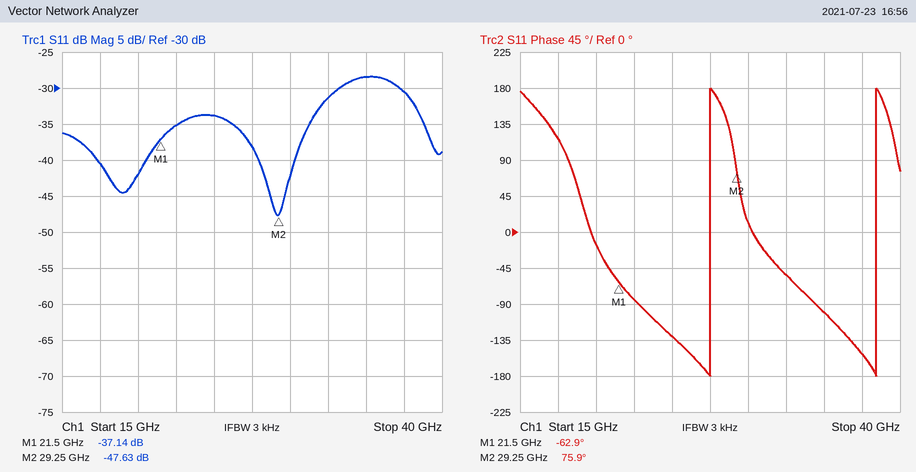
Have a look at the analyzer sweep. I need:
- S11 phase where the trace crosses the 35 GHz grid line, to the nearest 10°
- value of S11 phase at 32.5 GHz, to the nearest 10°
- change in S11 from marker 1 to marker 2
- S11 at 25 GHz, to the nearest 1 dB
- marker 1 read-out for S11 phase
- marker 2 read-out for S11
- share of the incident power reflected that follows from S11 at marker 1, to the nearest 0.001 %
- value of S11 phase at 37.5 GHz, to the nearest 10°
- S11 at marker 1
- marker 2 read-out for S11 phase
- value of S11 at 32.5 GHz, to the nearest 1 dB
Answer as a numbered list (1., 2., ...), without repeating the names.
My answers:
1. -100°
2. -50°
3. -10.49 dB
4. -34 dB
5. -62.9°
6. -47.63 dB
7. 0.019 %
8. -150°
9. -37.14 dB
10. 75.9°
11. -31 dB
